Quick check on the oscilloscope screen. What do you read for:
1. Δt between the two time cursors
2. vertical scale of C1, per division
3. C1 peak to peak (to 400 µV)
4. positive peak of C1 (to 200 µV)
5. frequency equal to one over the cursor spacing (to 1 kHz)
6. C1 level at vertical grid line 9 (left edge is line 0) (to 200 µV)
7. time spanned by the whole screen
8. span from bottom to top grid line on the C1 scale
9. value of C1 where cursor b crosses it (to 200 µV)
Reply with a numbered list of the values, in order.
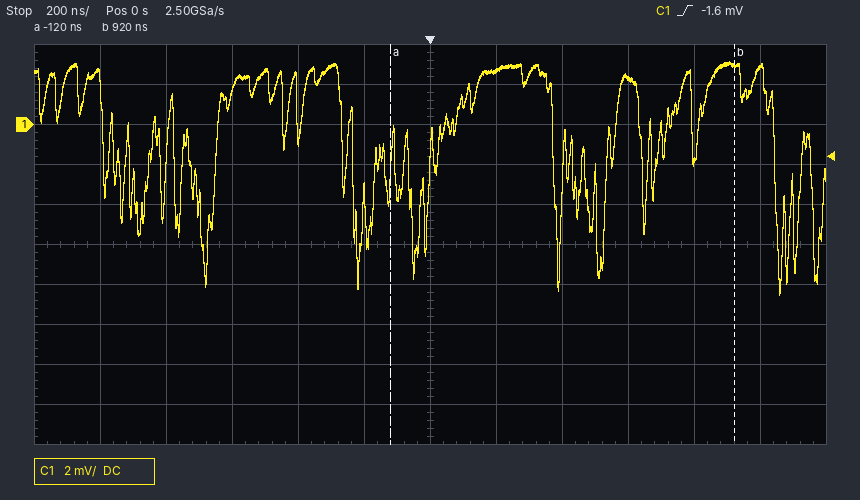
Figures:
1. 1.04 µs
2. 2 mV
3. 11.6 mV
4. 3.2 mV
5. 962 kHz
6. 2.4 mV
7. 2.4 µs
8. 20 mV
9. 3.0 mV
